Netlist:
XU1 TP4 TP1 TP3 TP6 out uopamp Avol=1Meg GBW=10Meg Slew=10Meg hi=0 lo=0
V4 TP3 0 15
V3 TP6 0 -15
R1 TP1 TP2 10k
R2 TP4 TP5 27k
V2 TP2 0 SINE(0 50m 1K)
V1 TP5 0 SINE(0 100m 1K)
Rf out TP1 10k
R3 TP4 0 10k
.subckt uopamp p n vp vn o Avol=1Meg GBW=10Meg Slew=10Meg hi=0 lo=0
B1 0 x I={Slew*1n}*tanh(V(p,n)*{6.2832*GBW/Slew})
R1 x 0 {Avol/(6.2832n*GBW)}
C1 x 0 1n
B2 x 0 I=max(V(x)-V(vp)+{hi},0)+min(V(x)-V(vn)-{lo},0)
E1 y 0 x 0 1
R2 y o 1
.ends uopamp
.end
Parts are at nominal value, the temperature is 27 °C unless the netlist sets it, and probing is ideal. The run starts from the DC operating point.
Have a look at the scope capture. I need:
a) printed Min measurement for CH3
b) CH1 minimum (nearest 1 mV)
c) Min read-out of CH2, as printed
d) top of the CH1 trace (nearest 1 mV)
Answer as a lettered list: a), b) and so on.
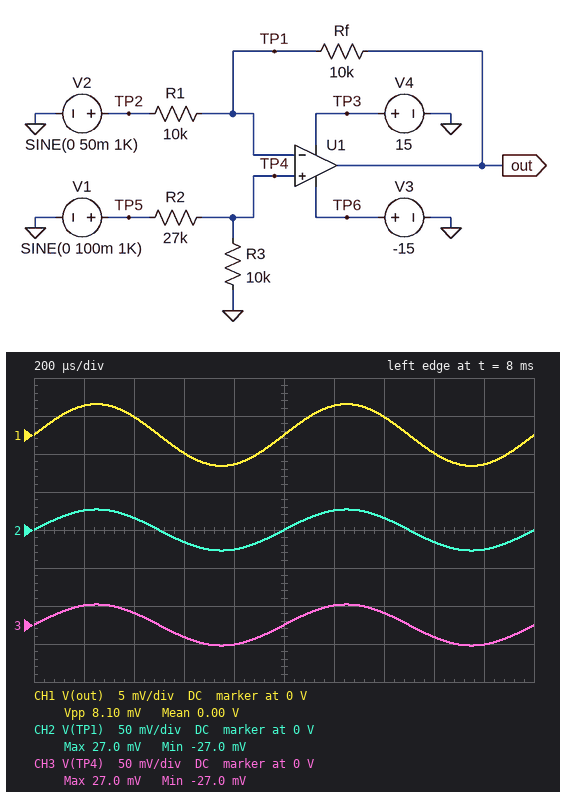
a) -27.0 mV
b) -4 mV
c) -27.0 mV
d) 4 mV
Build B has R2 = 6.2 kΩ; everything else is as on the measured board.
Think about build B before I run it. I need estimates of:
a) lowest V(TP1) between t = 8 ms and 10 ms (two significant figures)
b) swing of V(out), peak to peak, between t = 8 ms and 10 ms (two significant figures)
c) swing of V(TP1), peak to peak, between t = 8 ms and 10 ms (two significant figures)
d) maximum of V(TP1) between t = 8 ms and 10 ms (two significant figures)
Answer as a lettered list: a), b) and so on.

a) -62 mV
b) 150 mV
c) 120 mV
d) 62 mV
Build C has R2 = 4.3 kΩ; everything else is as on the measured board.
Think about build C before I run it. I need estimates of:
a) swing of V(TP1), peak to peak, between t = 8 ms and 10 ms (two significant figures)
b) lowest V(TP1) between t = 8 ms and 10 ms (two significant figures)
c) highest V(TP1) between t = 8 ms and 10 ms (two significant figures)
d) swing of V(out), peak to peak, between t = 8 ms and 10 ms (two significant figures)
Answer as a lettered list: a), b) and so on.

a) 140 mV
b) -70 mV
c) 70 mV
d) 180 mV
